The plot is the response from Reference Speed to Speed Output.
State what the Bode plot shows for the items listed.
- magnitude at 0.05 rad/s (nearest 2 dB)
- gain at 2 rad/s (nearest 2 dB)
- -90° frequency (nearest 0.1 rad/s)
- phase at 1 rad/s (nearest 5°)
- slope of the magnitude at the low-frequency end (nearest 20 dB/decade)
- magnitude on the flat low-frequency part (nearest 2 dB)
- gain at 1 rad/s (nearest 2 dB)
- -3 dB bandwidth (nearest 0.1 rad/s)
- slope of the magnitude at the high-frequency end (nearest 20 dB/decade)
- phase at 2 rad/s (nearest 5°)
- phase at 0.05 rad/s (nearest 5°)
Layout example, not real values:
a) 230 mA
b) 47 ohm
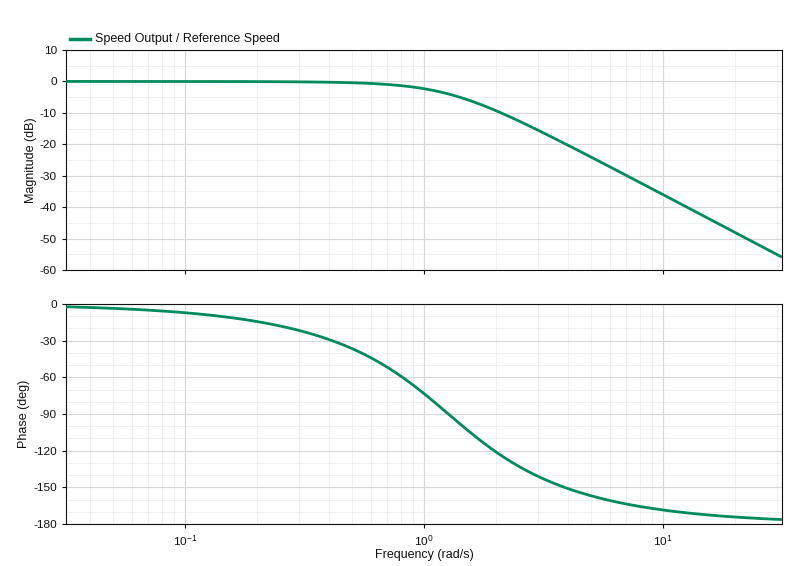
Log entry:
a) 0 dB
b) -10 dB
c) 1.3 rad/s
d) -75°
e) 0 dB/decade
f) 0 dB
g) -2 dB
h) 1.1 rad/s
i) -40 dB/decade
j) -120°
k) -5°
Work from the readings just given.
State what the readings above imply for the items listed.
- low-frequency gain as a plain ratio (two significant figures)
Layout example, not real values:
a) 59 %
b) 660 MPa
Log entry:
a) 1.0
